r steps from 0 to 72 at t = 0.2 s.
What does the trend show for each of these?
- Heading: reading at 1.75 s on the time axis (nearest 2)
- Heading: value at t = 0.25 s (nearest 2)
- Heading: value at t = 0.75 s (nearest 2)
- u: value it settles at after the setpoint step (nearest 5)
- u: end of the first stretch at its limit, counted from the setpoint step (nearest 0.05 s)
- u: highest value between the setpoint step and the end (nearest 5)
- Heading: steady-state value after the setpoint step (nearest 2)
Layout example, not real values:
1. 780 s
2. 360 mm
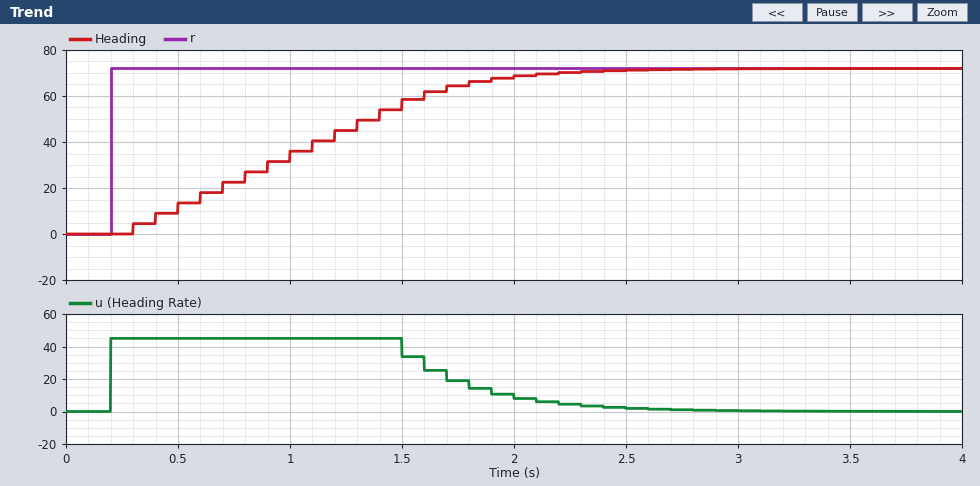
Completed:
1. 64
2. 0
3. 22
4. 0
5. 1.30 s
6. 45
7. 72
